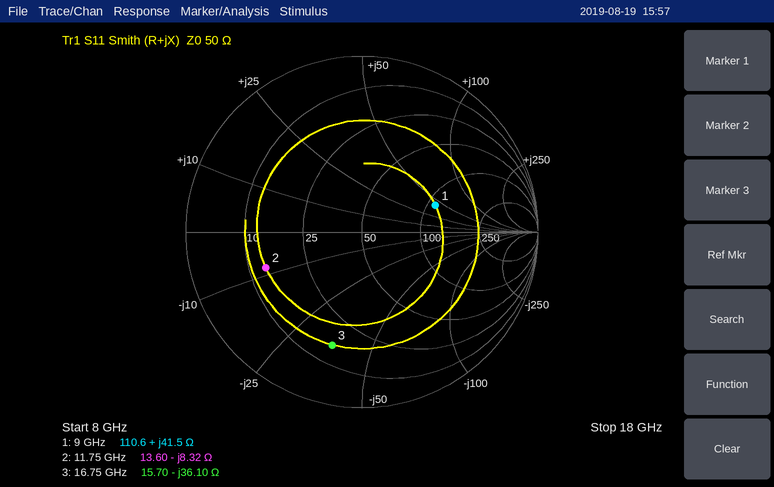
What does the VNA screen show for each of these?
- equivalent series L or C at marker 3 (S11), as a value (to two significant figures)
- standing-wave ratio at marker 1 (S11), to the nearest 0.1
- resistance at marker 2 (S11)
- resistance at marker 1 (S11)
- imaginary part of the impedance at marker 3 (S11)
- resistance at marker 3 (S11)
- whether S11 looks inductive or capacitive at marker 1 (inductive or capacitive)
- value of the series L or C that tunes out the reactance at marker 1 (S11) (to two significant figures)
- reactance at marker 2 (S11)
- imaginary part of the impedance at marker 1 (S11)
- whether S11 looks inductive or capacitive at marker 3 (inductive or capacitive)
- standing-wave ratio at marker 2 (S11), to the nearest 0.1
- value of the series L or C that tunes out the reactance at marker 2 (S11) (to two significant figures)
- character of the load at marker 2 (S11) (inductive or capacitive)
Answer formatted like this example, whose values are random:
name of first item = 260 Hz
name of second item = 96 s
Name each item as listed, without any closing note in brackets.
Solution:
equivalent series L or C at marker 3 (S11), as a value = 260 fF
standing-wave ratio at marker 1 (S11), to the nearest 0.1 = 2.6
resistance at marker 2 = 13.60 Ω
resistance at marker 1 = 110.6 Ω
imaginary part of the impedance at marker 3 = -36.10 Ω
resistance at marker 3 = 15.70 Ω
whether S11 looks inductive or capacitive at marker 1 = inductive
value of the series L or C that tunes out the reactance at marker 1 (S11) = 430 fF
reactance at marker 2 = -8.32 Ω
imaginary part of the impedance at marker 1 = +41.5 Ω
whether S11 looks inductive or capacitive at marker 3 = capacitive
standing-wave ratio at marker 2 (S11), to the nearest 0.1 = 3.8
value of the series L or C that tunes out the reactance at marker 2 (S11) = 110 pH
character of the load at marker 2 (S11) = capacitive
